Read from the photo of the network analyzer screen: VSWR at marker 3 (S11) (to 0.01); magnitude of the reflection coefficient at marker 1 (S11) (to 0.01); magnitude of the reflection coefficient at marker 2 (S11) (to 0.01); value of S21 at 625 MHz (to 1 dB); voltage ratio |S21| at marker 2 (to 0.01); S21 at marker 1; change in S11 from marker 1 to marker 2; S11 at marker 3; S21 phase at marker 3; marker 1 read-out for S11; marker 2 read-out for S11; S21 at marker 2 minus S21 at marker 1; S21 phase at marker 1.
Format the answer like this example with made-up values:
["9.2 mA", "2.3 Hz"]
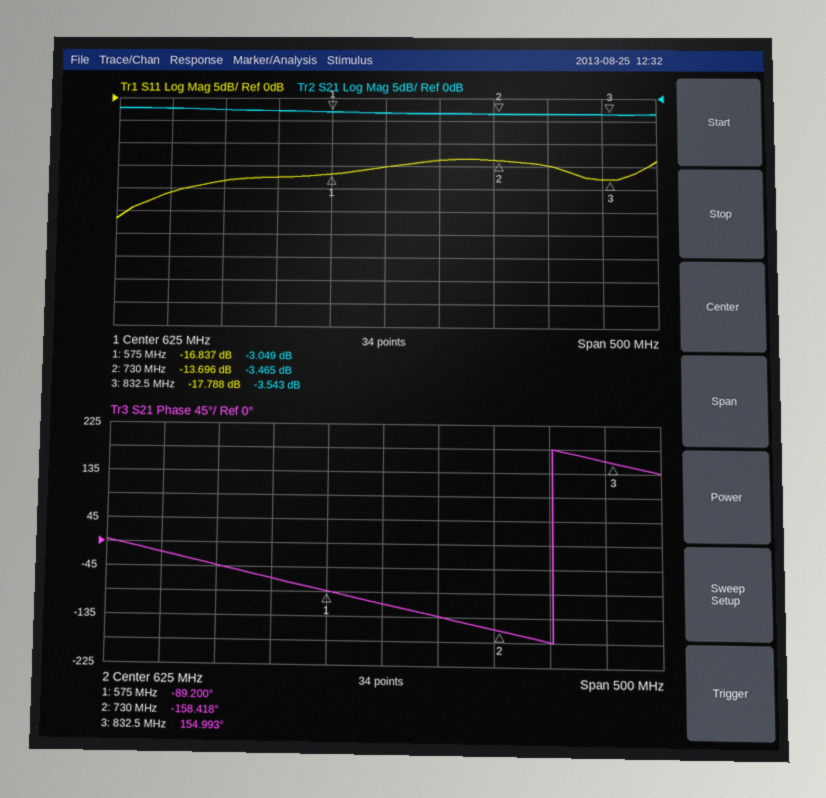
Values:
["1.30", "0.14", "0.21", "-3 dB", "0.67", "-3.049 dB", "3.141 dB", "-17.788 dB", "154.993°", "-16.837 dB", "-13.696 dB", "-0.416 dB", "-89.200°"]
